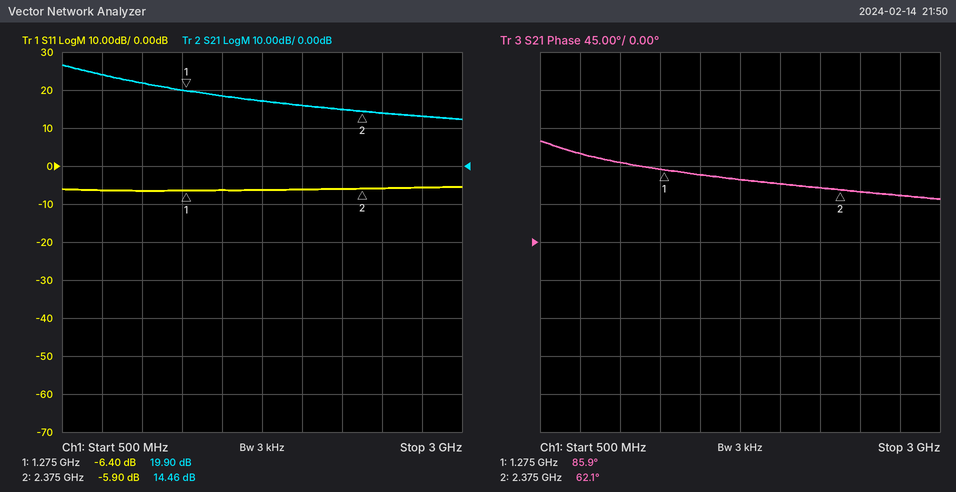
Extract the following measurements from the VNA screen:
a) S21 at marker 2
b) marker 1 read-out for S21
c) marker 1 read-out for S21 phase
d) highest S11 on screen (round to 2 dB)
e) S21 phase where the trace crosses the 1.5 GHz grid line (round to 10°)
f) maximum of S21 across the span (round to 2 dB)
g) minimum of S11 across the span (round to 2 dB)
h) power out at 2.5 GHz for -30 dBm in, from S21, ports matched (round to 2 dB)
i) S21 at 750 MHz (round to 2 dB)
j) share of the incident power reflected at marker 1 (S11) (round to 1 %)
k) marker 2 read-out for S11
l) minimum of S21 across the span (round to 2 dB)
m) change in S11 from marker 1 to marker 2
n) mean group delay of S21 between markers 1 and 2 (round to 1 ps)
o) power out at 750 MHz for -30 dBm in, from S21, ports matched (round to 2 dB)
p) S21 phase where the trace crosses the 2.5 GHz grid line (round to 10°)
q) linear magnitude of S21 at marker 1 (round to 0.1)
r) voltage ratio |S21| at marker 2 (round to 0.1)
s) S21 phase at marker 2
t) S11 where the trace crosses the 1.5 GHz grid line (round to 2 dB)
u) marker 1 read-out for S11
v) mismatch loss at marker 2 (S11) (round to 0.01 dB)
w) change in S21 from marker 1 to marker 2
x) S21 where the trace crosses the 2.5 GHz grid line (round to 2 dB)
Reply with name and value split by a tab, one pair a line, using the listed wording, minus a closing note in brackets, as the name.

S21 at marker 2	14.46 dB
marker 1 read-out for S21	19.90 dB
marker 1 read-out for S21 phase	85.9°
highest S11 on screen	-6 dB
S21 phase where the trace crosses the 1.5 GHz grid line	80°
maximum of S21 across the span	26 dB
minimum of S11 across the span	-6 dB
power out at 2.5 GHz for -30 dBm in, from S21, ports matched	-16 dBm
S21 at 750 MHz	24 dB
share of the incident power reflected at marker 1 (S11)	23 %
marker 2 read-out for S11	-5.90 dB
minimum of S21 across the span	12 dB
change in S11 from marker 1 to marker 2	0.50 dB
mean group delay of S21 between markers 1 and 2	60 ps
power out at 750 MHz for -30 dBm in, from S21, ports matched	-6 dBm
S21 phase where the trace crosses the 2.5 GHz grid line	60°
linear magnitude of S21 at marker 1	9.9
voltage ratio |S21| at marker 2	5.3
S21 phase at marker 2	62.1°
S11 where the trace crosses the 1.5 GHz grid line	-6 dB
marker 1 read-out for S11	-6.40 dB
mismatch loss at marker 2 (S11)	1.29 dB
change in S21 from marker 1 to marker 2	-5.44 dB
S21 where the trace crosses the 2.5 GHz grid line	14 dB
